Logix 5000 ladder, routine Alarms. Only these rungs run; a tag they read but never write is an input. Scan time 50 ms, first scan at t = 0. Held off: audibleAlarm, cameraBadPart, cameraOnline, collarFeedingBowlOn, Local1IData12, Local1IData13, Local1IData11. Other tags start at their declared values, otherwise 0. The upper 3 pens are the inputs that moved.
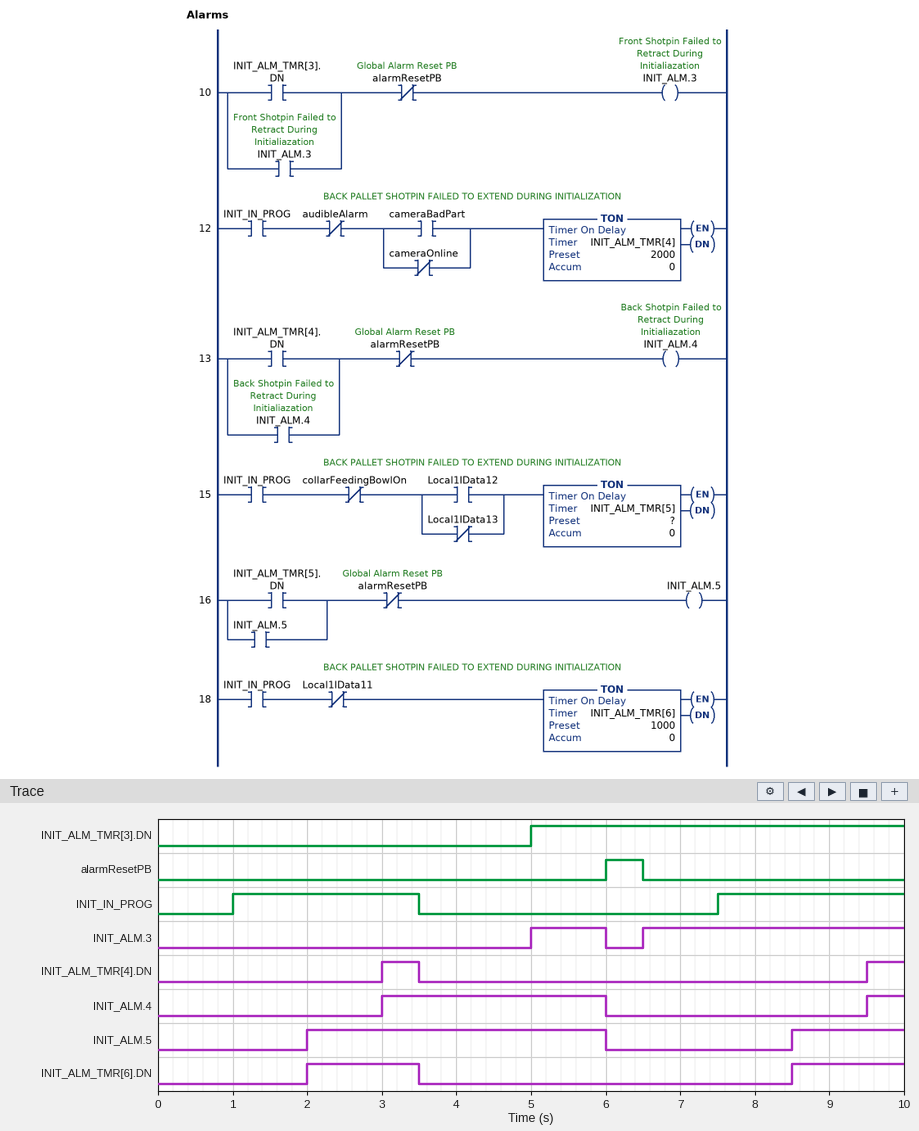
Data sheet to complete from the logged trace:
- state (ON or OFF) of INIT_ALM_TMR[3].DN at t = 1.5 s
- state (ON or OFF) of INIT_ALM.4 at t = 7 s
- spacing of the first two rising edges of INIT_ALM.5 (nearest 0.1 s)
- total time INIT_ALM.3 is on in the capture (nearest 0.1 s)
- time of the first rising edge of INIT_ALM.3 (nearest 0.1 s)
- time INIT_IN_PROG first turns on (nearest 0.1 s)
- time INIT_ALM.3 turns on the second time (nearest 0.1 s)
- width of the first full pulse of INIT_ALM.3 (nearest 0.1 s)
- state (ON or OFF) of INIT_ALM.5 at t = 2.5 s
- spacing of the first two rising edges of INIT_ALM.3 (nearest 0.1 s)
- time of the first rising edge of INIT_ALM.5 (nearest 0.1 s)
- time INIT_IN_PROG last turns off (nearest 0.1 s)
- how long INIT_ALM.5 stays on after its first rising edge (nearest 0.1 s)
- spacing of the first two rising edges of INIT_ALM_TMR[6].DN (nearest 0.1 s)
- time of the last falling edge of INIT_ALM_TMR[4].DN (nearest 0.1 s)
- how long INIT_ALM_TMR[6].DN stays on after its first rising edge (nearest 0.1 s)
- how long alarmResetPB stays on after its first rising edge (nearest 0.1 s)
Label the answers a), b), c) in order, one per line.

a) OFF
b) OFF
c) 6.5 s
d) 4.5 s
e) 5.0 s
f) 1.0 s
g) 6.5 s
h) 1.0 s
i) ON
j) 1.5 s
k) 2.0 s
l) 3.5 s
m) 4.0 s
n) 6.5 s
o) 3.5 s
p) 1.5 s
q) 0.5 s
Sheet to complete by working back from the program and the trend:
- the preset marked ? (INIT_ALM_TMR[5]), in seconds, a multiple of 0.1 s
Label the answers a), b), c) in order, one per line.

a) 1.0 s
